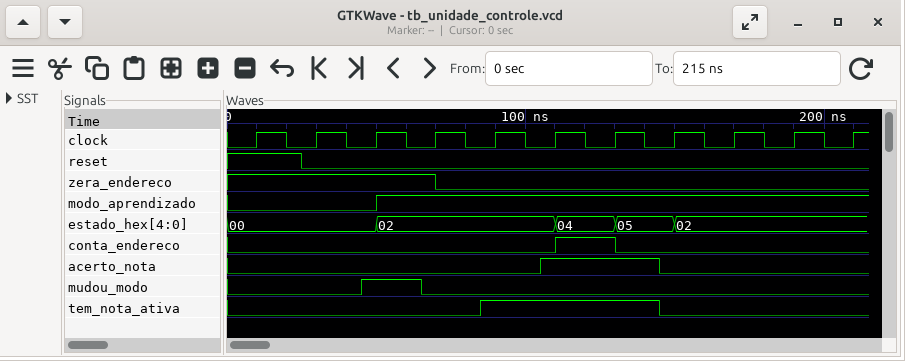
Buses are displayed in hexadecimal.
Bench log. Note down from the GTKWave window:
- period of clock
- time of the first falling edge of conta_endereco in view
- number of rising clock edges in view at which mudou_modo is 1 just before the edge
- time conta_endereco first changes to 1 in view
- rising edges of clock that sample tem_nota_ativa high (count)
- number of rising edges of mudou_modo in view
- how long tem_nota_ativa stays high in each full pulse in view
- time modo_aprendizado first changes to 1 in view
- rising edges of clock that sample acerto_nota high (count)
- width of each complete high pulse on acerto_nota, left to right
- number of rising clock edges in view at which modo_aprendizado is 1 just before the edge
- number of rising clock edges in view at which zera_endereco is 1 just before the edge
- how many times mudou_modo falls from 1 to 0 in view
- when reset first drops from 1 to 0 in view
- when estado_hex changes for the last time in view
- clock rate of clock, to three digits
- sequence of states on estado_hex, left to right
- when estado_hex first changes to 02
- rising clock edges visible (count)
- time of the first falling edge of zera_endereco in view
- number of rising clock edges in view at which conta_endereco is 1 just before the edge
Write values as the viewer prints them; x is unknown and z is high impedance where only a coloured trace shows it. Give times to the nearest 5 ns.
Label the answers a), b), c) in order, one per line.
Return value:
a) 20 ns
b) 130 ns
c) 1
d) 110 ns
e) 3
f) 1
g) 60 ns
h) 50 ns
i) 2
j) 40 ns
k) 8
l) 4
m) 1
n) 25 ns
o) 150 ns
p) 50.0 MHz
q) 00, 02, 04, 05, 02
r) 50 ns
s) 11
t) 70 ns
u) 1
